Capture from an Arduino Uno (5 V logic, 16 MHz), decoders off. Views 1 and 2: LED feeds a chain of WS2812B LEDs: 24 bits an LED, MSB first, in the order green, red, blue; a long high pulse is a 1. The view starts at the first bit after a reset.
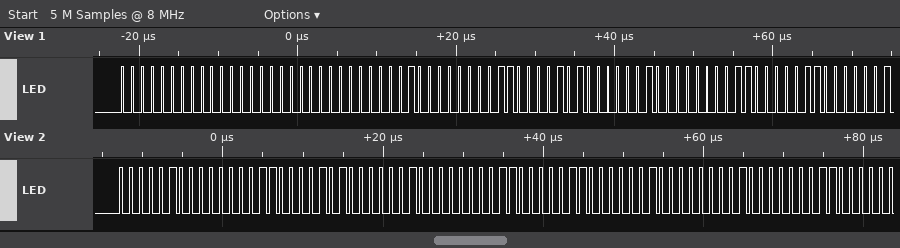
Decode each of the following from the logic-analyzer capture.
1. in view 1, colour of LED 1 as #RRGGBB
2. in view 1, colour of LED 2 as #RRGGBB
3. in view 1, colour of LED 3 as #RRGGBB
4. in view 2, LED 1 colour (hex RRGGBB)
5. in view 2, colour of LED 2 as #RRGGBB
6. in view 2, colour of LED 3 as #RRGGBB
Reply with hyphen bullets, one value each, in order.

- #000000
- #03040A
- #030406
- #03040A
- #030406
- #020403
